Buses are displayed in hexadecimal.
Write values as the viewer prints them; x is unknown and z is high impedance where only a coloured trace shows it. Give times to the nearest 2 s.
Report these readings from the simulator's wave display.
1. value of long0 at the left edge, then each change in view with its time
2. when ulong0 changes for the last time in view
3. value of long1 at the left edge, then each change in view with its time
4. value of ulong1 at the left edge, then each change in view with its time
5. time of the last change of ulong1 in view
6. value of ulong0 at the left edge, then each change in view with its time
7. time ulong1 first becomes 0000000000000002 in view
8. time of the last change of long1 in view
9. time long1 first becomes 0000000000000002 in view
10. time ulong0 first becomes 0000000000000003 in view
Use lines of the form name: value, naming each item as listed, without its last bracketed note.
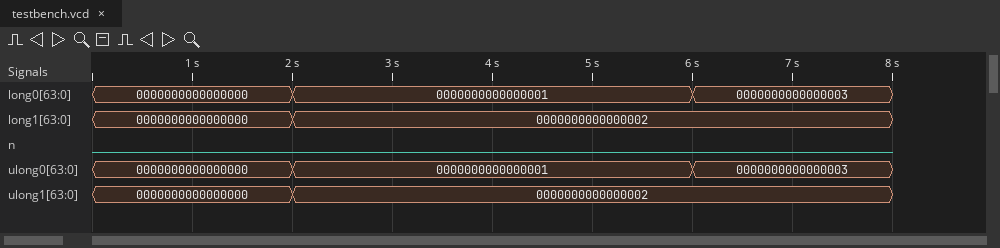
value of long0 at the left edge, then each change in view with its time: 0000000000000000, 0000000000000001 at 2 s, 0000000000000003 at 6 s
when ulong0 changes for the last time in view: 6 s
value of long1 at the left edge, then each change in view with its time: 0000000000000000, 0000000000000002 at 2 s
value of ulong1 at the left edge, then each change in view with its time: 0000000000000000, 0000000000000002 at 2 s
time of the last change of ulong1 in view: 2 s
value of ulong0 at the left edge, then each change in view with its time: 0000000000000000, 0000000000000001 at 2 s, 0000000000000003 at 6 s
time ulong1 first becomes 0000000000000002 in view: 2 s
time of the last change of long1 in view: 2 s
time long1 first becomes 0000000000000002 in view: 2 s
time ulong0 first becomes 0000000000000003 in view: 6 s
